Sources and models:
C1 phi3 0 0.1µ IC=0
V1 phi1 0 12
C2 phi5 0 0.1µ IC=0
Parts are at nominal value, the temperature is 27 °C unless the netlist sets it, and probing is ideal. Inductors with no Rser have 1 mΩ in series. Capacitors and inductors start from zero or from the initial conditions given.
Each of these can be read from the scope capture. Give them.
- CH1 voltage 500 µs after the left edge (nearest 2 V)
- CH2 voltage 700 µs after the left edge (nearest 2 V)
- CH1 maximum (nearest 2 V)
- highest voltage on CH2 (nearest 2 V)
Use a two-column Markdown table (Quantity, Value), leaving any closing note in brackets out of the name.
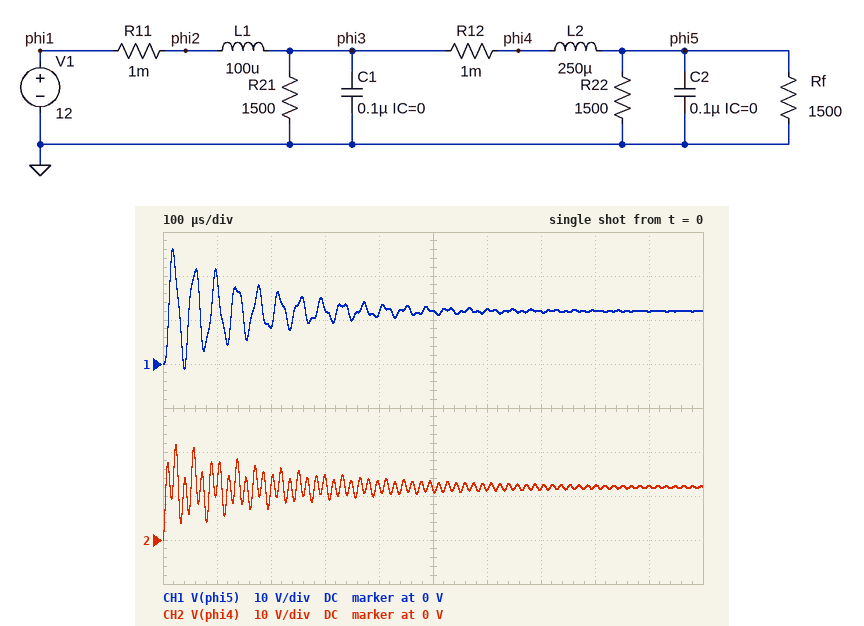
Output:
| Quantity | Value |
|---|---|
| CH1 voltage 500 µs after the left edge | 12 V |
| CH2 voltage 700 µs after the left edge | 12 V |
| CH1 maximum | 26 V |
| highest voltage on CH2 | 22 V |
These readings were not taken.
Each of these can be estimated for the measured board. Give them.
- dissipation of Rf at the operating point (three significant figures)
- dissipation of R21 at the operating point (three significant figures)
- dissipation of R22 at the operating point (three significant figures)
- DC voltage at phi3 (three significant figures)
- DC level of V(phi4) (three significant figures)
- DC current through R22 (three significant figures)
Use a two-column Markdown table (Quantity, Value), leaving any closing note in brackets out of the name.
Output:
| Quantity | Value |
|---|---|
| dissipation of Rf at the operating point | 96.0 mW |
| dissipation of R21 at the operating point | 96.0 mW |
| dissipation of R22 at the operating point | 96.0 mW |
| DC voltage at phi3 | 12.0 V |
| DC level of V(phi4) | 12.0 V |
| DC current through R22 | 8.00 mA |
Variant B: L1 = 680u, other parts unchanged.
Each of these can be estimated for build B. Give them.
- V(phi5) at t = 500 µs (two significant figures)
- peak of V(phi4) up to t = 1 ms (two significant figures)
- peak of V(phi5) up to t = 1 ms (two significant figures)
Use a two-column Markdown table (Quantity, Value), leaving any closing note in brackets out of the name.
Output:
| Quantity | Value |
|---|---|
| V(phi5) at t = 500 µs | 13 V |
| peak of V(phi4) up to t = 1 ms | 21 V |
| peak of V(phi5) up to t = 1 ms | 23 V |
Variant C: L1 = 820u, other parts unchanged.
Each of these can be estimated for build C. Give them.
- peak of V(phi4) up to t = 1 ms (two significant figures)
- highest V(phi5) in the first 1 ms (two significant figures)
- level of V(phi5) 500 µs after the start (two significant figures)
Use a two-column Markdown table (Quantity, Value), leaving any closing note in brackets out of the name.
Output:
| Quantity | Value |
|---|---|
| peak of V(phi4) up to t = 1 ms | 20 V |
| highest V(phi5) in the first 1 ms | 23 V |
| level of V(phi5) 500 µs after the start | 11 V |
